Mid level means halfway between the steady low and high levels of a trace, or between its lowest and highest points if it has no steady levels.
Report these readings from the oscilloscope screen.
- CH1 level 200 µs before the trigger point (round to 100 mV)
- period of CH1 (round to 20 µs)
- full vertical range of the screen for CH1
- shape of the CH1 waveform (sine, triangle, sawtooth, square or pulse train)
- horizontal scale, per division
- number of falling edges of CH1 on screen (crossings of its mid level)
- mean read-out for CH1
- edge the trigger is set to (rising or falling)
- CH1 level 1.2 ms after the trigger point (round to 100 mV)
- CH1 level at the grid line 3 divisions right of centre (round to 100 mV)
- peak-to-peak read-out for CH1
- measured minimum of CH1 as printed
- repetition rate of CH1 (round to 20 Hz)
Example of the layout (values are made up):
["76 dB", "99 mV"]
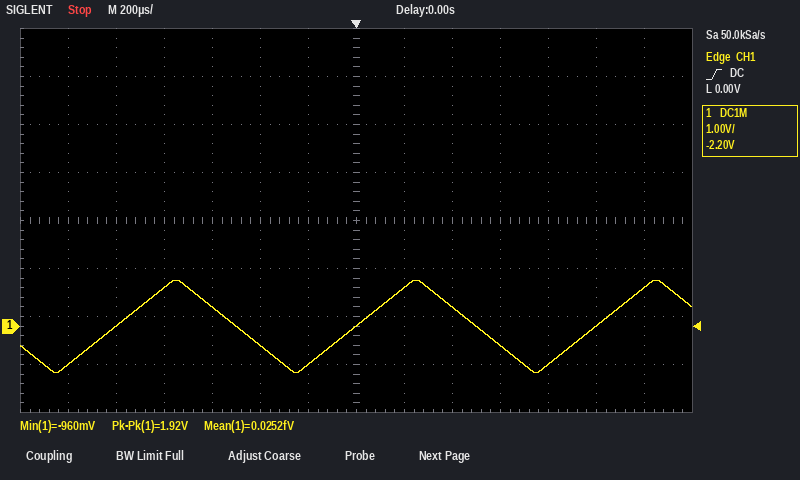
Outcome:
["-800 mV", "1.00 ms", "8 V", "triangle", "200 µs", "2", "0.0252 fV", "rising", "800 mV", "-400 mV", "1.92 V", "-960 mV", "1.00 kHz"]
